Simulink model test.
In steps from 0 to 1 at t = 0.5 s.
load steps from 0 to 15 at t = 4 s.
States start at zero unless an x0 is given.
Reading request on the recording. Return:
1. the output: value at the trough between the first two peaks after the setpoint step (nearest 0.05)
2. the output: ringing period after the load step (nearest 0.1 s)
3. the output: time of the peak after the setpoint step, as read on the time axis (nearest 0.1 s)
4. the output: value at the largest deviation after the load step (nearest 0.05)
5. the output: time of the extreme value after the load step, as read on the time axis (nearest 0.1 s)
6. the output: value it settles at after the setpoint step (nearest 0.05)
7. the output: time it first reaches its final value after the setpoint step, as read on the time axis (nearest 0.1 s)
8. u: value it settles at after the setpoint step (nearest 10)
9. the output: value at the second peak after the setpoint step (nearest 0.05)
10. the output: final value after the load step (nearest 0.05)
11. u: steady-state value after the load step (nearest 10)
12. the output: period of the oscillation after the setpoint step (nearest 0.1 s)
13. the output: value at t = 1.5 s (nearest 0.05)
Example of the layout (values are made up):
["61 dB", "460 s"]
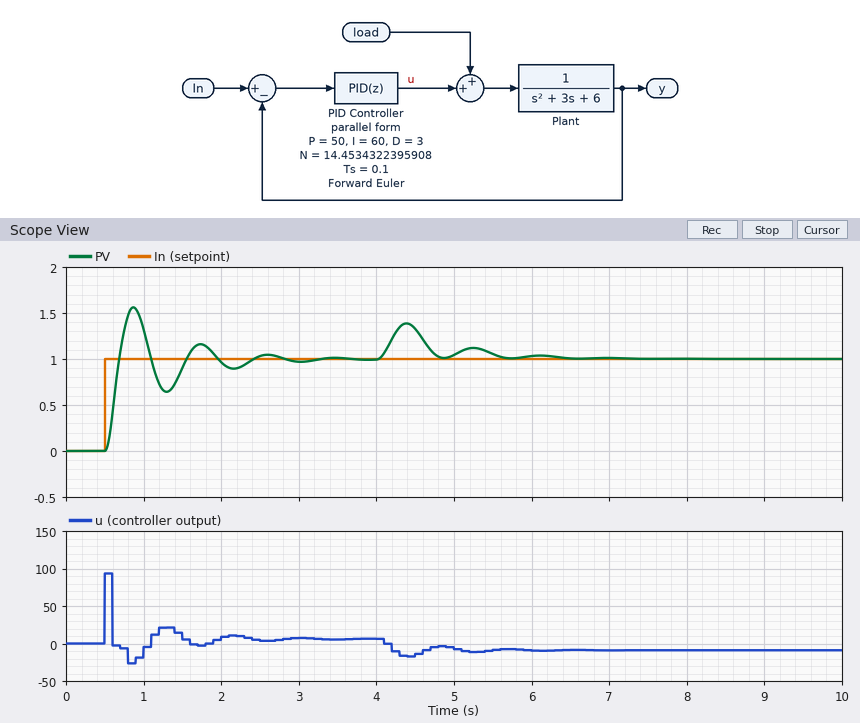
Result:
["0.65", "0.9 s", "0.9 s", "1.40", "4.4 s", "1.00", "0.7 s", "10", "1.15", "1.00", "-10", "0.9 s", "0.90"]
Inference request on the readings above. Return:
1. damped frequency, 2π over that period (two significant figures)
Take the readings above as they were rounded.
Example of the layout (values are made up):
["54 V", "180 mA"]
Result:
["7.0 rad/s"]
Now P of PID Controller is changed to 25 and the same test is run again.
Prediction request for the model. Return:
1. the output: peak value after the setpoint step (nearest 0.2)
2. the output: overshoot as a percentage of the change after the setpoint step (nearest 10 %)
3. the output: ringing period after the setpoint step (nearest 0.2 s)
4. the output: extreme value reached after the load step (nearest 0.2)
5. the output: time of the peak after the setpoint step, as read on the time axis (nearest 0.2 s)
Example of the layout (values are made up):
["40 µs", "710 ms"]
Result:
["1.4", "40 %", "1.4 s", "1.6", "1.0 s"]
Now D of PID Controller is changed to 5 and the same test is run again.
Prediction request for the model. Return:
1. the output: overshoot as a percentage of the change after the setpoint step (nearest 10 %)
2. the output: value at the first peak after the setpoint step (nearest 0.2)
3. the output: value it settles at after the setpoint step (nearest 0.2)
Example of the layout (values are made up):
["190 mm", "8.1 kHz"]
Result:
["40 %", "1.4", "1.0"]
